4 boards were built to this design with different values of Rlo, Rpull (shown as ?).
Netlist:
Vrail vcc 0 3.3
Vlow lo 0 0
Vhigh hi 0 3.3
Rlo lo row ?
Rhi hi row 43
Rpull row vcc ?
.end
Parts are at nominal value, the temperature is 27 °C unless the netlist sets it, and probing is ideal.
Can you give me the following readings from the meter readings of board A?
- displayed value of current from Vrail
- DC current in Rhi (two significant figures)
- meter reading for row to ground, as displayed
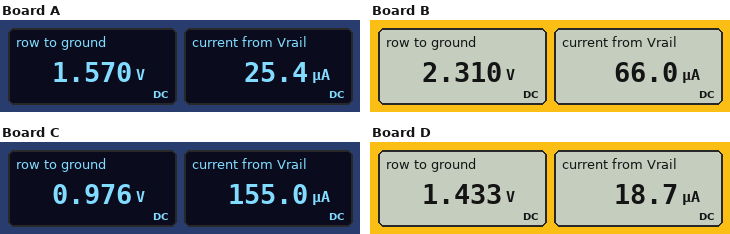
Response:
25.4 µA
40 mA
1.570 V
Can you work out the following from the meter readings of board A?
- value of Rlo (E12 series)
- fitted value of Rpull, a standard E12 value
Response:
39 Ω
68 kΩ
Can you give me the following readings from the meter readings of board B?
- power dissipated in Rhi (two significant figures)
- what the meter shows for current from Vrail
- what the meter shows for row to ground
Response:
23 mW
66.0 µA
2.310 V
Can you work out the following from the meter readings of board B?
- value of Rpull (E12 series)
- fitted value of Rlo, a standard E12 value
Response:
15 kΩ
100 Ω
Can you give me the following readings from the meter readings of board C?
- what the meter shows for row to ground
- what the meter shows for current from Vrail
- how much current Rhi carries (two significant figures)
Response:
0.976 V
155.0 µA
54 mA
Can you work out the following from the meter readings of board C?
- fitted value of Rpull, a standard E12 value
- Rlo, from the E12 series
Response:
15 kΩ
18 Ω
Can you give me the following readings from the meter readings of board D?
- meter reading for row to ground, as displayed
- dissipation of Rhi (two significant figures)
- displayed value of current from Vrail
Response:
1.433 V
81 mW
18.7 µA
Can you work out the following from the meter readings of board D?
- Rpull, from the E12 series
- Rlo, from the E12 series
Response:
100 kΩ
33 Ω
